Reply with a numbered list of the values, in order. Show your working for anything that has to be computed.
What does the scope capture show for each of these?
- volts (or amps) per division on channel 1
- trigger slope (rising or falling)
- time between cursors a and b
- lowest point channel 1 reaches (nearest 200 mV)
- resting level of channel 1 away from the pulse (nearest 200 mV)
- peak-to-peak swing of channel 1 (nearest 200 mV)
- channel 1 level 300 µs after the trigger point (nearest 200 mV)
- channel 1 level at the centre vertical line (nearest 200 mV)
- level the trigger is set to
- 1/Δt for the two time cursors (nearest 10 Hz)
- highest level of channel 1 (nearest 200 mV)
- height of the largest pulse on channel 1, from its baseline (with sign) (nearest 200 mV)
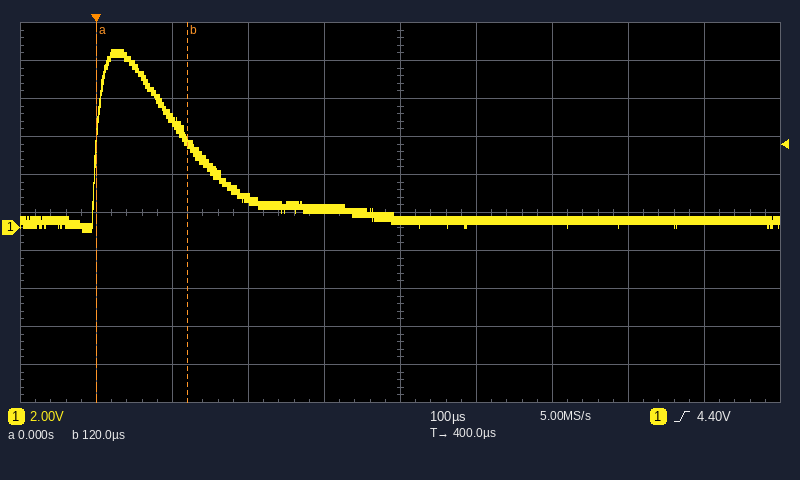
1. 2 V
2. rising
3. 120 µs − (0 s) = 120 µs
4. -200 mV
5. 400 mV
6. 9.4 V − (-200 mV) = 9.6 V
7. 1.0 V
8. 400 mV
9. 4.40 V
10. 1 / 120 µs ≈ 8.33 kHz
11. 9.4 V
12. 9.4 V − (400 mV) = +9.0 V
